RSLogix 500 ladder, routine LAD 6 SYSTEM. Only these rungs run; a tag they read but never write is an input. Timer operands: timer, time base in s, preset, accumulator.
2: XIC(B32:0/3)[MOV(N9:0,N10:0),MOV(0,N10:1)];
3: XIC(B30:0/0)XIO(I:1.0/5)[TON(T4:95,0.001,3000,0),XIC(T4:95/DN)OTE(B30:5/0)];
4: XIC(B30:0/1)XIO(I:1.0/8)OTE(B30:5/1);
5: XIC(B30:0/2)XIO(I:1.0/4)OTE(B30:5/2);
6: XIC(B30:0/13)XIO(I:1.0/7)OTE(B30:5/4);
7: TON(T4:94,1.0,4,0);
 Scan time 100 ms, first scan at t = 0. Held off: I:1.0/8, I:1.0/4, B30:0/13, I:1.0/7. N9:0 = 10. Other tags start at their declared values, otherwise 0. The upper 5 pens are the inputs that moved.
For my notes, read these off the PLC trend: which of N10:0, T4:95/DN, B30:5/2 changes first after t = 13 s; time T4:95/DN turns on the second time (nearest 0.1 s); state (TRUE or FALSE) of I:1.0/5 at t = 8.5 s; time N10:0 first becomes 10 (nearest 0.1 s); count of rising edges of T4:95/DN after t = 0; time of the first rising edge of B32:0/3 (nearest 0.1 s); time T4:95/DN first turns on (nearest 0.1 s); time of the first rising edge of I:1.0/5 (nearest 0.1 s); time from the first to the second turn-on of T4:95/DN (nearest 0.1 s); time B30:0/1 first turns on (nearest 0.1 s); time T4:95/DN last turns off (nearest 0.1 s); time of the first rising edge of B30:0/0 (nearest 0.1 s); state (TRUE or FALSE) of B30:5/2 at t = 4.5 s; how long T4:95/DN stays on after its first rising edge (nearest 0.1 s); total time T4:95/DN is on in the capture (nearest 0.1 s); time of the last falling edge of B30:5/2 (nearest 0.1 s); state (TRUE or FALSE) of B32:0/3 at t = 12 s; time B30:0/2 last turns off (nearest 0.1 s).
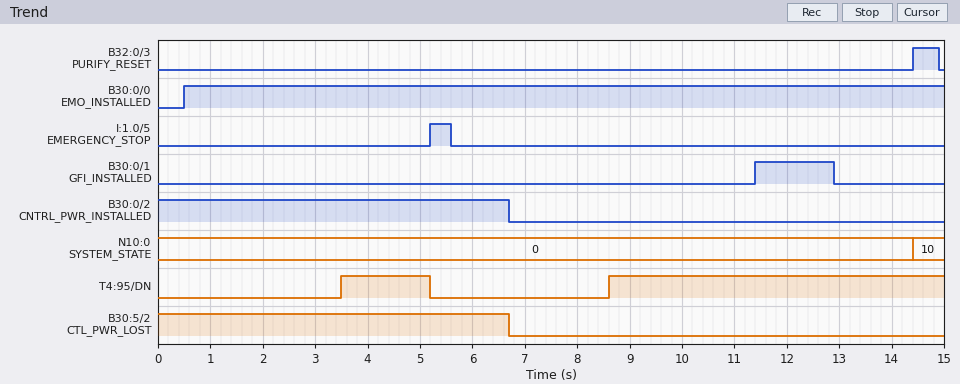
N10:0
8.6 s
FALSE
14.4 s
2
14.4 s
3.5 s
5.2 s
5.1 s
11.4 s
5.2 s
0.5 s
TRUE
1.7 s
8.1 s
6.7 s
FALSE
6.7 s
